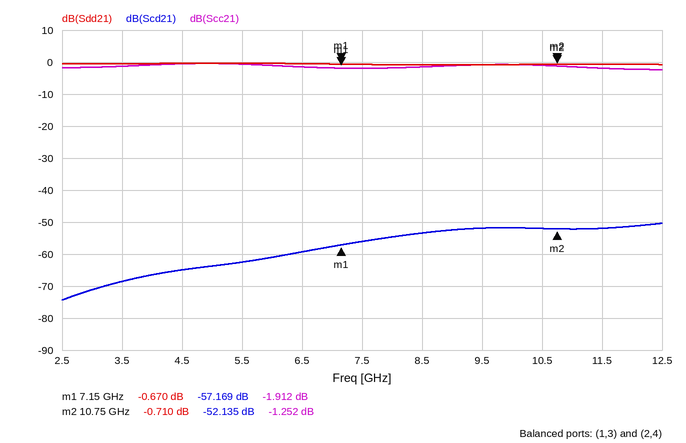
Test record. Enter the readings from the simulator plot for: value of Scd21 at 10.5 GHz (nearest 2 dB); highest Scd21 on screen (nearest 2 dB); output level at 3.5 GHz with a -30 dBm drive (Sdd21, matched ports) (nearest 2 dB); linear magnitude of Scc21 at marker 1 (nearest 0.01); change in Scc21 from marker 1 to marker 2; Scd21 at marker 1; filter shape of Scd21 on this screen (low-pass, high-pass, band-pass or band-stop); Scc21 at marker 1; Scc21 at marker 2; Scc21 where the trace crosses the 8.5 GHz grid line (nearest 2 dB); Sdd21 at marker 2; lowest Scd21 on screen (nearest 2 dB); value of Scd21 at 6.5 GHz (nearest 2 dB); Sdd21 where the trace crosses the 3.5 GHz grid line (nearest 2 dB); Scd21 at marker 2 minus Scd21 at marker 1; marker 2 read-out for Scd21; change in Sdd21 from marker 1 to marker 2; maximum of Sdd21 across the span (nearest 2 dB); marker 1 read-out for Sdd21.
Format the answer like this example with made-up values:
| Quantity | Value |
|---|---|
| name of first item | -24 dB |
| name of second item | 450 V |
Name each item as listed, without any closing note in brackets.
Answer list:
| Quantity | Value |
|---|---|
| value of Scd21 at 10.5 GHz | -52 dB |
| highest Scd21 on screen | -50 dB |
| output level at 3.5 GHz with a -30 dBm drive (Sdd21, matched ports) | -30 dBm |
| linear magnitude of Scc21 at marker 1 | 0.80 |
| change in Scc21 from marker 1 to marker 2 | 0.660 dB |
| Scd21 at marker 1 | -57.169 dB |
| filter shape of Scd21 on this screen | high-pass |
| Scc21 at marker 1 | -1.912 dB |
| Scc21 at marker 2 | -1.252 dB |
| Scc21 where the trace crosses the 8.5 GHz grid line | -2 dB |
| Sdd21 at marker 2 | -0.710 dB |
| lowest Scd21 on screen | -74 dB |
| value of Scd21 at 6.5 GHz | -60 dB |
| Sdd21 where the trace crosses the 3.5 GHz grid line | 0 dB |
| Scd21 at marker 2 minus Scd21 at marker 1 | 5.034 dB |
| marker 2 read-out for Scd21 | -52.135 dB |
| change in Sdd21 from marker 1 to marker 2 | -0.040 dB |
| maximum of Sdd21 across the span | 0 dB |
| marker 1 read-out for Sdd21 | -0.670 dB |
